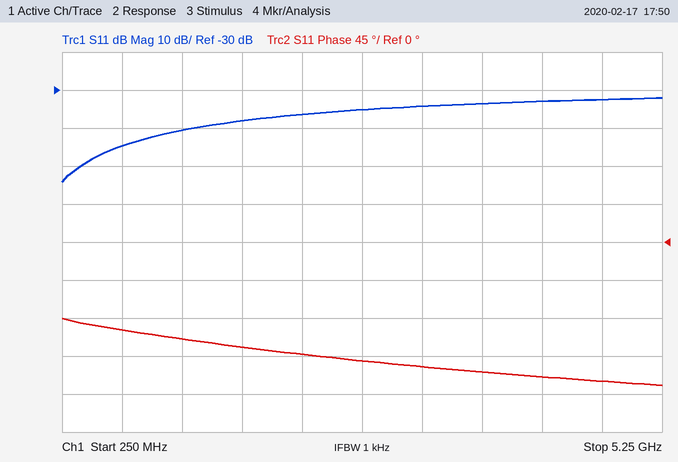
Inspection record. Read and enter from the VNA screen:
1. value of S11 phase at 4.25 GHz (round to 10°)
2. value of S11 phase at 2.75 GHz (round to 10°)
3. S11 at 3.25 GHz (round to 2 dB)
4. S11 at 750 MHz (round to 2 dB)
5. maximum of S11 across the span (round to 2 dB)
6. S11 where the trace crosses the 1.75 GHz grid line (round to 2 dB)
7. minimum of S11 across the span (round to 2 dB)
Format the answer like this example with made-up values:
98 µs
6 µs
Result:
-160°
-140°
-34 dB
-44 dB
-32 dB
-38 dB
-54 dB
